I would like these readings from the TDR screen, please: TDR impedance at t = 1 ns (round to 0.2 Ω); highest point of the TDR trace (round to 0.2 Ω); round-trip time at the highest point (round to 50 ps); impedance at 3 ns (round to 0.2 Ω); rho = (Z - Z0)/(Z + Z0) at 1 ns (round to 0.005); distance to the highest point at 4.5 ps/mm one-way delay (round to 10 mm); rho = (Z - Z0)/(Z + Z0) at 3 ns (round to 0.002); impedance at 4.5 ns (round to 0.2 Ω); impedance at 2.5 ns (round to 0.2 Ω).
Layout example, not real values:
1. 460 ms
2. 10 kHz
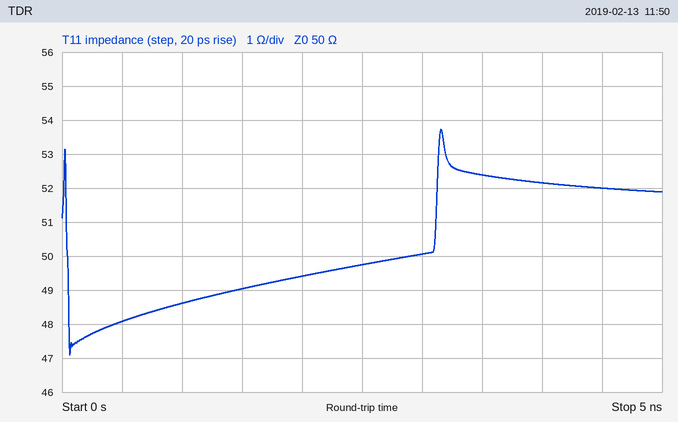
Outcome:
1. 48.6 Ω
2. 53.8 Ω
3. 3.15 ns
4. 50.0 Ω
5. -0.015
6. 350 mm
7. 0.000
8. 52.0 Ω
9. 49.8 Ω
